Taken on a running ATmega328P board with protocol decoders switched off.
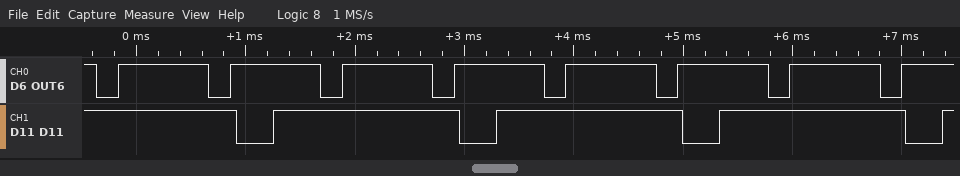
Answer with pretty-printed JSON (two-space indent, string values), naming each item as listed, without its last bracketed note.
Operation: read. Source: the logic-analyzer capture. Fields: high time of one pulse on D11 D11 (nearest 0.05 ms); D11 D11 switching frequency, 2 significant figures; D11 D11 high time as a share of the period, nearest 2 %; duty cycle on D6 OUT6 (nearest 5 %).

{
  "high time of one pulse on D11 D11": "1.70 ms",
  "D11 D11 switching frequency, 2 significant figures": "490 Hz",
  "D11 D11 high time as a share of the period, nearest 2 %": "84 %",
  "duty cycle on D6 OUT6": "80 %"
}
